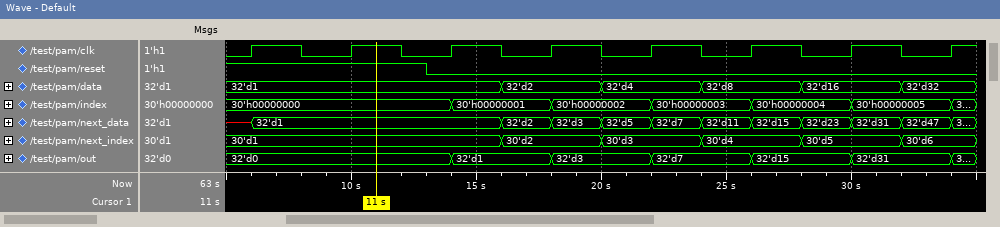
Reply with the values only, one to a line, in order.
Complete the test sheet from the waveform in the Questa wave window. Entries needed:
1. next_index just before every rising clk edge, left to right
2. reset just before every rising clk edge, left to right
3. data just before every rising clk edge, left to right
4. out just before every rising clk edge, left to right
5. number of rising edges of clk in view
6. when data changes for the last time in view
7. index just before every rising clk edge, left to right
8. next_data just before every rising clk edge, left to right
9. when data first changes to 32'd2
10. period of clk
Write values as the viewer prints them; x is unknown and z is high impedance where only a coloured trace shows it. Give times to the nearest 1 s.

30'd1, 30'd1, 30'd1, 30'd2, 30'd3, 30'd4, 30'd5, 30'd6
1 1 0 0 0 0 0 0
32'd1, 32'd1, 32'd1, 32'd2, 32'd4, 32'd8, 32'd16, 32'd32
32'd0, 32'd0, 32'd0, 32'd1, 32'd3, 32'd7, 32'd15, 32'd31
8
32 s
30'h00000000, 30'h00000000, 30'h00000000, 30'h00000001, 30'h00000002, 30'h00000003, 30'h00000004, 30'h00000005
x, 32'd1, 32'd1, 32'd2, 32'd5, 32'd11, 32'd23, 32'd47
16 s
4 s
